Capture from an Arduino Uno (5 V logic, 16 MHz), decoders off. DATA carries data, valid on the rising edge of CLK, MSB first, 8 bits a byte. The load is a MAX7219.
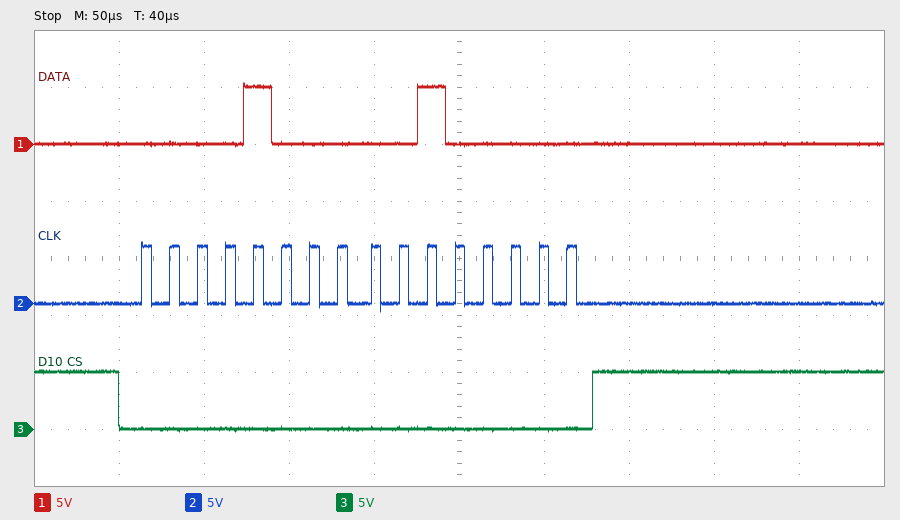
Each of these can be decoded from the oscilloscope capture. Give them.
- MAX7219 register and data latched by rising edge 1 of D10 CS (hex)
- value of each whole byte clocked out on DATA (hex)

register 0x8, data 0x20
08 20
